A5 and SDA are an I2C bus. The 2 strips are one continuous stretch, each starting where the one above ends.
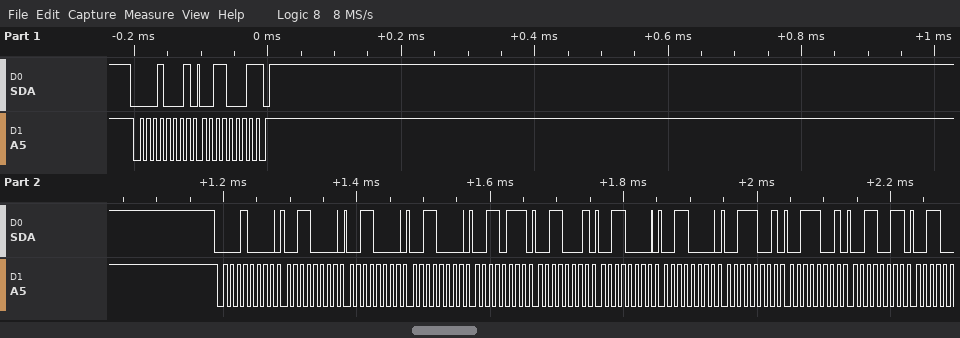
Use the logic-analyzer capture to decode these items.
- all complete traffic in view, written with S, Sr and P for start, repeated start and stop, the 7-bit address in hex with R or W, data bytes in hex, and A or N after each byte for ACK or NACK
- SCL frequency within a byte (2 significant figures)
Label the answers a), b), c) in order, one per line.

a) S 08R A 31 N P S 08W A 30 A 30 A 30 A 37 A 31 A 30 A 30 A 39 A 39 A 33 A
b) 100 kHz
